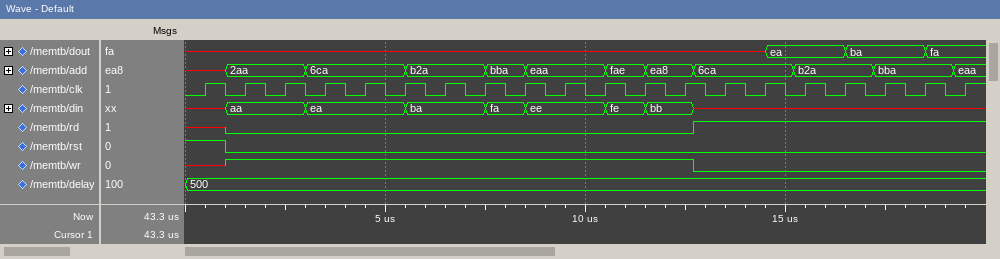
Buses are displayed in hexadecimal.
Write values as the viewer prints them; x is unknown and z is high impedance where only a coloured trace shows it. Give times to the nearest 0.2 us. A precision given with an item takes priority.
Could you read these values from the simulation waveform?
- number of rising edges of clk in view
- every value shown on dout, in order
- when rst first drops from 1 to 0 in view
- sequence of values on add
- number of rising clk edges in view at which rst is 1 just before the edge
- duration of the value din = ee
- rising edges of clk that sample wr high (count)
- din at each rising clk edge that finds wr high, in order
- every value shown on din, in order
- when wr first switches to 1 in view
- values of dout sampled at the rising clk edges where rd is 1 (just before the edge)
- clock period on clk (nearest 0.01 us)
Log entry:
20
x, ea, ba, fa
1 us
x, 2aa, 6ca, b2a, bba, eaa, fae, ea8, 6ca, b2a, bba, eaa
1
2 us
12
aa, aa, ea, ea, ea, ba, ba, fa, ee, ee, fe, bb
x, aa, ea, ba, fa, ee, fe, bb, x
1 us
x, x, ea, ea, ba, ba, fa
1 us
